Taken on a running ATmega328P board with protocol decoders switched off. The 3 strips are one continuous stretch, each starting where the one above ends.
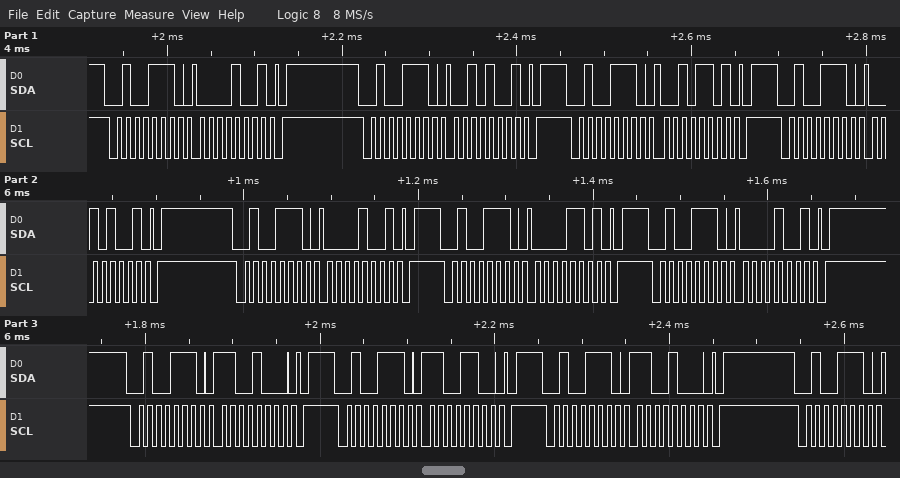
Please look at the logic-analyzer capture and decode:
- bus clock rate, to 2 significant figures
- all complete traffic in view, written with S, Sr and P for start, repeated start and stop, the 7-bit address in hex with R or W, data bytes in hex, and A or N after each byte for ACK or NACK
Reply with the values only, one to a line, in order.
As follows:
100 kHz
S 27W A 09 A P S 27W A 29 A P S 27W A 2D A P S 27W A 29 A P S 27W A 09 A P S 27W A 0D A P S 27W A 09 A P S 27W A C8 A P S 27W A CC A P S 27W A C8 A P S 27W A
